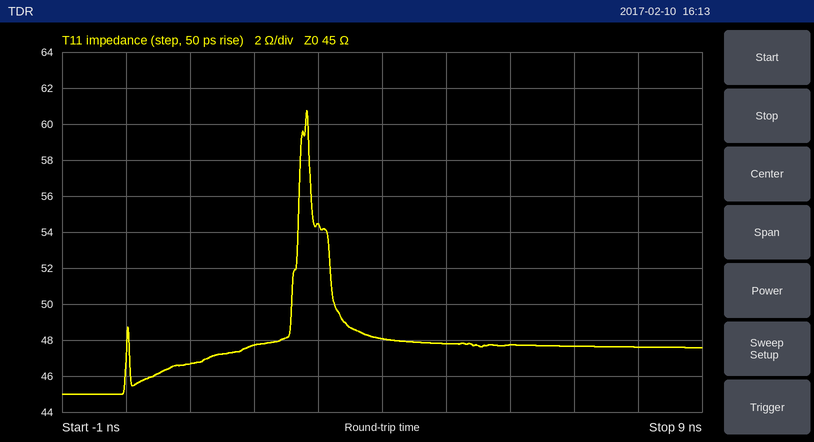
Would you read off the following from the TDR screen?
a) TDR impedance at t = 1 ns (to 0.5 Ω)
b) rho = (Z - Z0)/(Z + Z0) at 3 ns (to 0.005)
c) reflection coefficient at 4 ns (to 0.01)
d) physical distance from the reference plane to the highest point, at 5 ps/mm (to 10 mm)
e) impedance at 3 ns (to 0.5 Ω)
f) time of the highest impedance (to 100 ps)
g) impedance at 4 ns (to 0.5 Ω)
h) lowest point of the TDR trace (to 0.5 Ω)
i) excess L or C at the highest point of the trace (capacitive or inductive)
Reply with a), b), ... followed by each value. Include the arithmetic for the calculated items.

a) 46.5 Ω
b) (54.5 − 45)/(54.5 + 45) ≈ +0.095
c) (48 − 45)/(48 + 45) ≈ +0.03
d) 2.8 ns / 2 / 5 ps/mm ≈ 280 mm
e) 54.5 Ω
f) 2.8 ns
g) 48.0 Ω
h) 45.0 Ω
i) inductive
